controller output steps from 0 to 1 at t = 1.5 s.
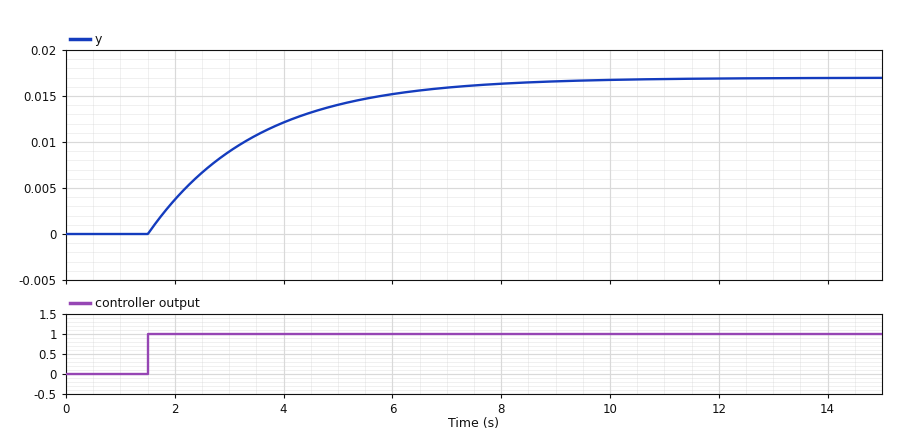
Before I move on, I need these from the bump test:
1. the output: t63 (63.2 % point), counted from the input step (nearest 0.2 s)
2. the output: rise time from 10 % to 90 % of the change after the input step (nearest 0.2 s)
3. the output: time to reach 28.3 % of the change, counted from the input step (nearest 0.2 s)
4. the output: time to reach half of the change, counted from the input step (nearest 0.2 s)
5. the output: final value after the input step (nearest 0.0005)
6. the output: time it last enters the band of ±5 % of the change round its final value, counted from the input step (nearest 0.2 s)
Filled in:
2.0 s
4.4 s
0.6 s
1.4 s
0.0170
6.0 s
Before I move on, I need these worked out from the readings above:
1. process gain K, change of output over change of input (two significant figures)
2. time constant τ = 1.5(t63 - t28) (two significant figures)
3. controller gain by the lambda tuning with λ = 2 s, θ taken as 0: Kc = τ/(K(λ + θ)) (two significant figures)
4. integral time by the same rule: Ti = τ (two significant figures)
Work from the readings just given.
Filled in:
0.017
2.1 s
62
2.1 s
